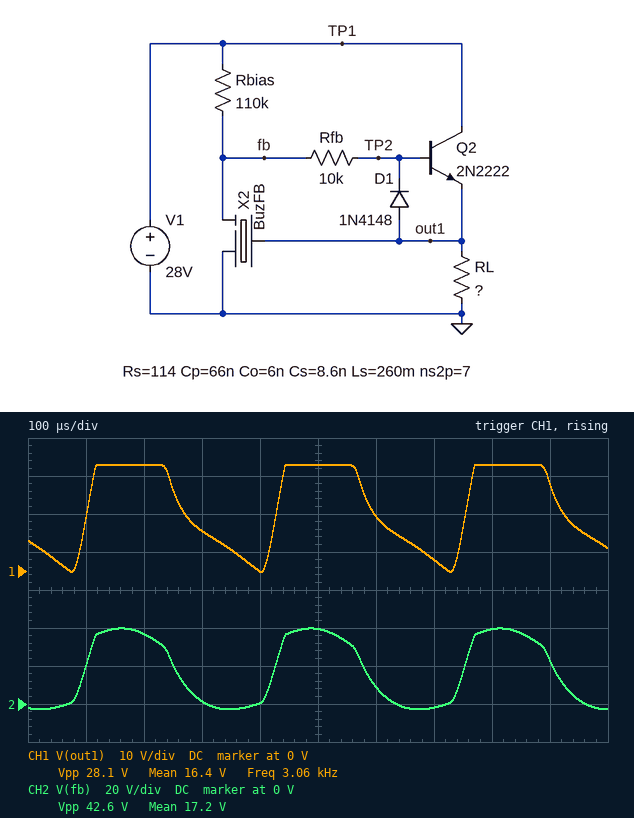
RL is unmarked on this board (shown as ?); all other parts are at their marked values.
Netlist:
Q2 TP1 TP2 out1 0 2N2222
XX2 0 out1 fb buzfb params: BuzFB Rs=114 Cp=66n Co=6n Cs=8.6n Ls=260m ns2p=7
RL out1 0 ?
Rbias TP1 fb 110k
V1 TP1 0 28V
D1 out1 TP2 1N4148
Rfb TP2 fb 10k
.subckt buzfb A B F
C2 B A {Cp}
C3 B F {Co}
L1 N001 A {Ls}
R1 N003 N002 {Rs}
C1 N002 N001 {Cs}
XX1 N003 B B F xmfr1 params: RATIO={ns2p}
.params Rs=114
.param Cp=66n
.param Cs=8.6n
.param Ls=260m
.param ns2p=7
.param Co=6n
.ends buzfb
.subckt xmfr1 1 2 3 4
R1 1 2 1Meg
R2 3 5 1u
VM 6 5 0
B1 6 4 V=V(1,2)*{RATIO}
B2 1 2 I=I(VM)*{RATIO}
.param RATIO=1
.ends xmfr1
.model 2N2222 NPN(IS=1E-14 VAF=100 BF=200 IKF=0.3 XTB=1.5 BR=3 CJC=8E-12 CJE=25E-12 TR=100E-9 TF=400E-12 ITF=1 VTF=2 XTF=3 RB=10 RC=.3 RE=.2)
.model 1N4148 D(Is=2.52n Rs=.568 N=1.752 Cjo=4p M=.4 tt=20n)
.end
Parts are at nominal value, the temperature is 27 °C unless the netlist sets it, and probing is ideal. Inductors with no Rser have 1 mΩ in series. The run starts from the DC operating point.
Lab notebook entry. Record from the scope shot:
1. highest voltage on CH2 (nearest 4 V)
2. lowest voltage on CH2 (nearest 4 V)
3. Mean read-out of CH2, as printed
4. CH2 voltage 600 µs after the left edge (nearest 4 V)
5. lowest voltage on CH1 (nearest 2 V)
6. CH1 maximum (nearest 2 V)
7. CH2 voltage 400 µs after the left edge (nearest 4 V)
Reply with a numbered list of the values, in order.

1. 40 V
2. -4 V
3. 17.2 V
4. 8 V
5. 0 V
6. 28 V
7. 0 V
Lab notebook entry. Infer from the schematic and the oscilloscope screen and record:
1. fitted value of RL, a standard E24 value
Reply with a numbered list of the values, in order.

1. 560 Ω
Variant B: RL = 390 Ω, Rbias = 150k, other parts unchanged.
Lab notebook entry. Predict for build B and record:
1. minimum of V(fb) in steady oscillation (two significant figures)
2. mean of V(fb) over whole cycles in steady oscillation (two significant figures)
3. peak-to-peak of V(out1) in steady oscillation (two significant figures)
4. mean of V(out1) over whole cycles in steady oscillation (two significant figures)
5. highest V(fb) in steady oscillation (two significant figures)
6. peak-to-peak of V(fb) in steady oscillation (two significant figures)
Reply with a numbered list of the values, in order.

1. -7.9 V
2. 16 V
3. 30 V
4. 15 V
5. 43 V
6. 51 V
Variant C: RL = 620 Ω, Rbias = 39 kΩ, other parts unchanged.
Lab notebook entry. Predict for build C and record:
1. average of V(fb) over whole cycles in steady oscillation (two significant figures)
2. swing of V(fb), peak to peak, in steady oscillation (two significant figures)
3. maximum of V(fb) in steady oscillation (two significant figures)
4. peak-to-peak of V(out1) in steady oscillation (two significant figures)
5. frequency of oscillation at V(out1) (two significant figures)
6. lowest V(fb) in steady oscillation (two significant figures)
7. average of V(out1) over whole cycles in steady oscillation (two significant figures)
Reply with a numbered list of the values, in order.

1. 21 V
2. 43 V
3. 43 V
4. 26 V
5. 3.2 kHz
6. -290 mV
7. 19 V
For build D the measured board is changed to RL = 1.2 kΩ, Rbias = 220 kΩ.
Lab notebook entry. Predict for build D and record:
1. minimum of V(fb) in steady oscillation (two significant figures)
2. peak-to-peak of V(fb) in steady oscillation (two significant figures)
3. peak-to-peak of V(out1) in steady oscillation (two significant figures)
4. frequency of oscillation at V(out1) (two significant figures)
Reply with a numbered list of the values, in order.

1. 3.6 V
2. 29 V
3. 25 V
4. 2.5 kHz
